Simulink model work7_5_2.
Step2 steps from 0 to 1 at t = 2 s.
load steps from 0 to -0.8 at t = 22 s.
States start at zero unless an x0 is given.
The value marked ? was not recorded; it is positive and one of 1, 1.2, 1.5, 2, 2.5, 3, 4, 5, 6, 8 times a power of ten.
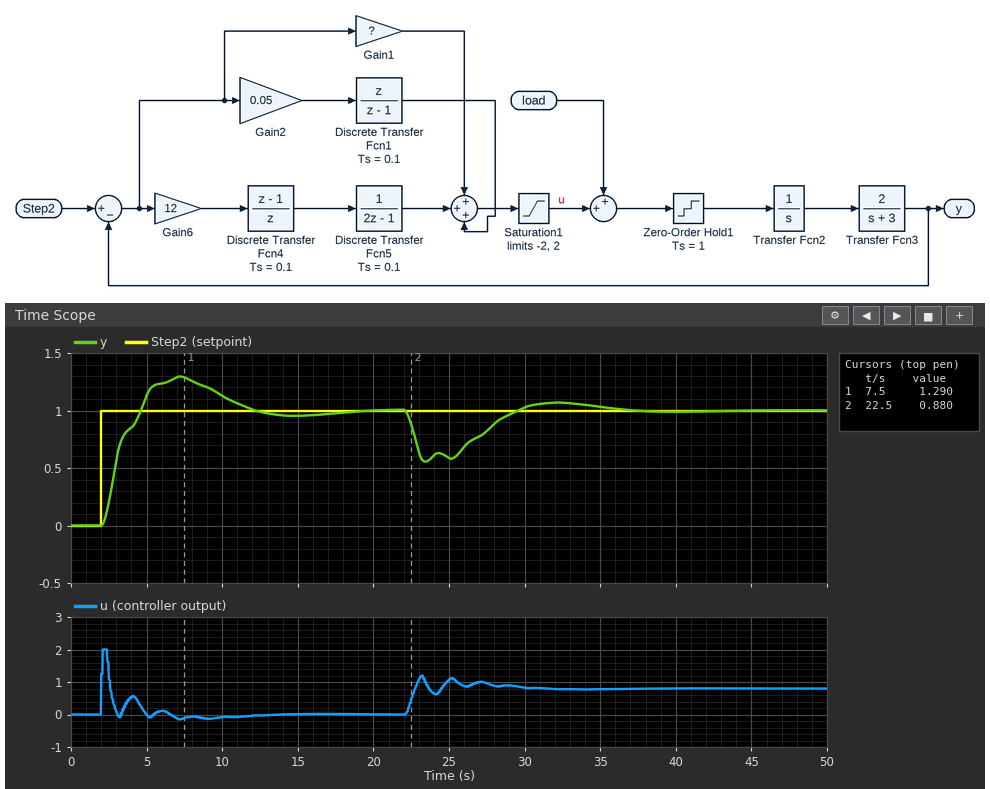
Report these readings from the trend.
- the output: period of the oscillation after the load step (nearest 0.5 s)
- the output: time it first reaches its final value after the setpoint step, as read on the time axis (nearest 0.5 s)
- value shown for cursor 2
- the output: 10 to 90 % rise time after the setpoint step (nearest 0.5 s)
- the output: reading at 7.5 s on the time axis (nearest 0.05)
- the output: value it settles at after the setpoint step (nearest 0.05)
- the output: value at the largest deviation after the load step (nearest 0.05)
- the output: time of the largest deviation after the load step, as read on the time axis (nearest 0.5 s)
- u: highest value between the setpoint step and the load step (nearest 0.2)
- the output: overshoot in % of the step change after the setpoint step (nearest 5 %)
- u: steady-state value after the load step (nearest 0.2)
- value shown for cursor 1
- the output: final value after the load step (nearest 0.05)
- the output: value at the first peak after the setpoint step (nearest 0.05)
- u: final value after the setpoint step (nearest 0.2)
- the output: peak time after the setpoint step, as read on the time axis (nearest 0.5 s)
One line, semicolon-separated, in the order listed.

1.5 s; 4.5 s; 0.880; 2.0 s; 1.30; 1.00; 0.55; 23.5 s; 2.0; 30 %; 0.8; 1.290; 1.00; 1.30; 0.0; 7.0 s
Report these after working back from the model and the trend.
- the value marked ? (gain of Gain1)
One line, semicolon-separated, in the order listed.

1.2
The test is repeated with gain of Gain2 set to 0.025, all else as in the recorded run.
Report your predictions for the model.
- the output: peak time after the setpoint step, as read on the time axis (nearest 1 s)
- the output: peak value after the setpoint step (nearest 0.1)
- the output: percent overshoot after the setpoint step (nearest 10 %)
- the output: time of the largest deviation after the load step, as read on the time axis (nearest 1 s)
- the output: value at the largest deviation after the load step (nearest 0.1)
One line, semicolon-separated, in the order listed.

9 s; 1.2; 20 %; 25 s; 0.5
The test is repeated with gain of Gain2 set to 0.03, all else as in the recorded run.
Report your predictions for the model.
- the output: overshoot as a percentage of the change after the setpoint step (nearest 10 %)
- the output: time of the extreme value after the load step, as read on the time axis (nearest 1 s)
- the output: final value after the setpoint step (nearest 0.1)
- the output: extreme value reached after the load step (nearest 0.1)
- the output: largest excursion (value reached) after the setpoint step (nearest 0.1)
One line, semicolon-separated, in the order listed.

20 %; 25 s; 1.0; 0.5; 1.2
